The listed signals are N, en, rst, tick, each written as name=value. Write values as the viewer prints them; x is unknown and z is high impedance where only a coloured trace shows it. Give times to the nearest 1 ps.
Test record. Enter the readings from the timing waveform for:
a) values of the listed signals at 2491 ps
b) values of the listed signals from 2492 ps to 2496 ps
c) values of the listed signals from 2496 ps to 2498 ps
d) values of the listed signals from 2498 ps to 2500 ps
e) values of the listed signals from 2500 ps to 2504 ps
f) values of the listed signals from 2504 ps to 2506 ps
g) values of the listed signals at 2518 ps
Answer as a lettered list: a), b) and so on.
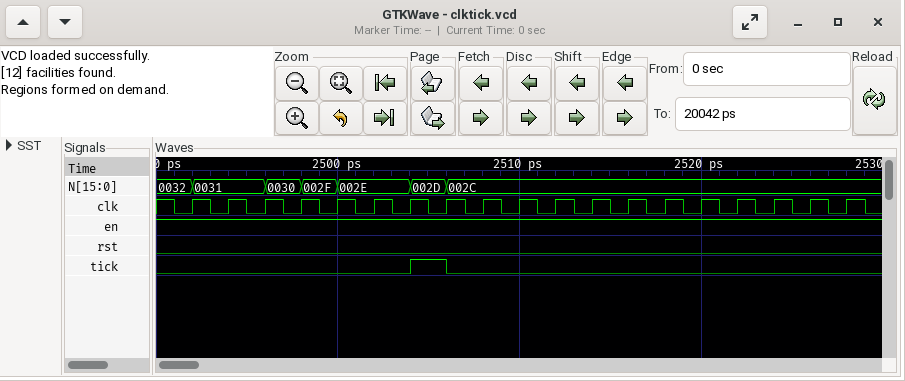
a) N=0032, en=1, rst=0, tick=0
b) N=0031, en=1, rst=0, tick=0
c) N=0030, en=1, rst=0, tick=0
d) N=002F, en=1, rst=0, tick=0
e) N=002E, en=1, rst=0, tick=0
f) N=002D, en=1, rst=0, tick=1
g) N=002C, en=1, rst=0, tick=0
